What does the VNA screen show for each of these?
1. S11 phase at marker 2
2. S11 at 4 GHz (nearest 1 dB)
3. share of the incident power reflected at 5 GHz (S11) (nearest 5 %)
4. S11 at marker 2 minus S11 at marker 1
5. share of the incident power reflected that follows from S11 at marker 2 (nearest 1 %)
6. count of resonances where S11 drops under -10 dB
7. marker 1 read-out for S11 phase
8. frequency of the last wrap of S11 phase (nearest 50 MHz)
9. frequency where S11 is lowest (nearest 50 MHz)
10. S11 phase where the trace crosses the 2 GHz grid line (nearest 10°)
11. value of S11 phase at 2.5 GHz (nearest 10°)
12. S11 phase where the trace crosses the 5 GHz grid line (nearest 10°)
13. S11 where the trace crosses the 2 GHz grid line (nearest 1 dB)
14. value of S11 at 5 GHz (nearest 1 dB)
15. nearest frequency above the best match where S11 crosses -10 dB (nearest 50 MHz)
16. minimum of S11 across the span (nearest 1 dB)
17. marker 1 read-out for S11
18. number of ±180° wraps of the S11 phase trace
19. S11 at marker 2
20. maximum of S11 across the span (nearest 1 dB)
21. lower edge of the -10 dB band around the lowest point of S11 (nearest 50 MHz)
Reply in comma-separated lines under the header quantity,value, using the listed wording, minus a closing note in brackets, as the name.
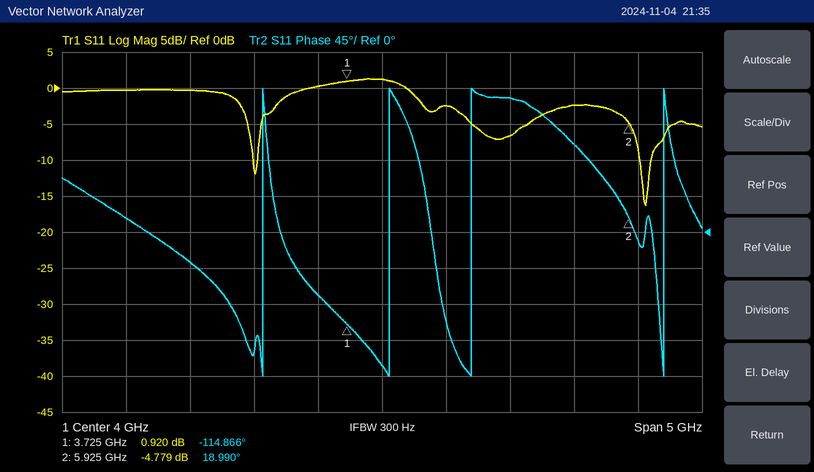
quantity,value
S11 phase at marker 2,18.990°
S11 at 4 GHz,1 dB
share of the incident power reflected at 5 GHz (S11),20 %
S11 at marker 2 minus S11 at marker 1,-5.699 dB
share of the incident power reflected that follows from S11 at marker 2,33 %
count of resonances where S11 drops under -10 dB,2
marker 1 read-out for S11 phase,-114.866°
frequency of the last wrap of S11 phase,6.20 GHz
frequency where S11 is lowest,6.05 GHz
S11 phase where the trace crosses the 2 GHz grid line,20°
value of S11 phase at 2.5 GHz,-40°
S11 phase where the trace crosses the 5 GHz grid line,170°
S11 where the trace crosses the 2 GHz grid line,0 dB
value of S11 at 5 GHz,-7 dB
nearest frequency above the best match where S11 crosses -10 dB,6.10 GHz
minimum of S11 across the span,-16 dB
marker 1 read-out for S11,0.920 dB
number of ±180° wraps of the S11 phase trace,4
S11 at marker 2,-4.779 dB
maximum of S11 across the span,1 dB
lower edge of the -10 dB band around the lowest point of S11,6.00 GHz
